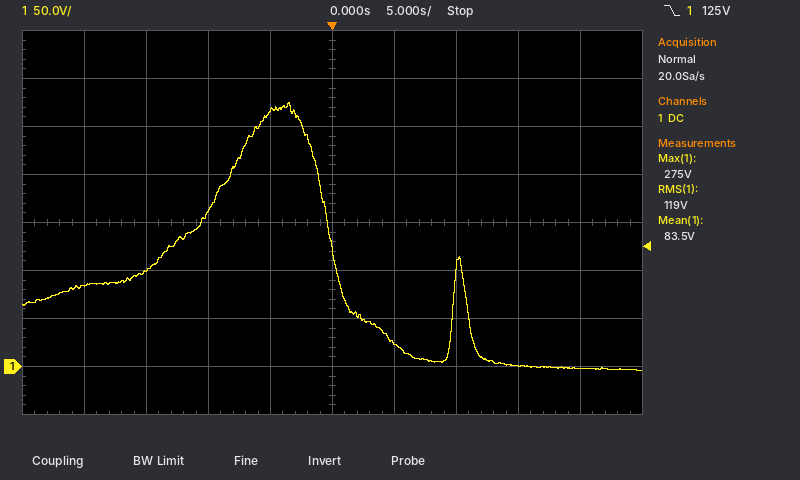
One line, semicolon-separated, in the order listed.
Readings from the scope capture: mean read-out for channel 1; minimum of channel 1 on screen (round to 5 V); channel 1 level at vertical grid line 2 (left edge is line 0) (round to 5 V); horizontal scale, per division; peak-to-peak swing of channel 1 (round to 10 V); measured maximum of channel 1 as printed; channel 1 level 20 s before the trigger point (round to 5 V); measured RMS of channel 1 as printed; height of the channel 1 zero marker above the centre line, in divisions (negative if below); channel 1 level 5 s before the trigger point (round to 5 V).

83.5 V; -5 V; 100 V; 5 s; 280 V; 275 V; 85 V; 119 V; -3.0 div; 265 V
